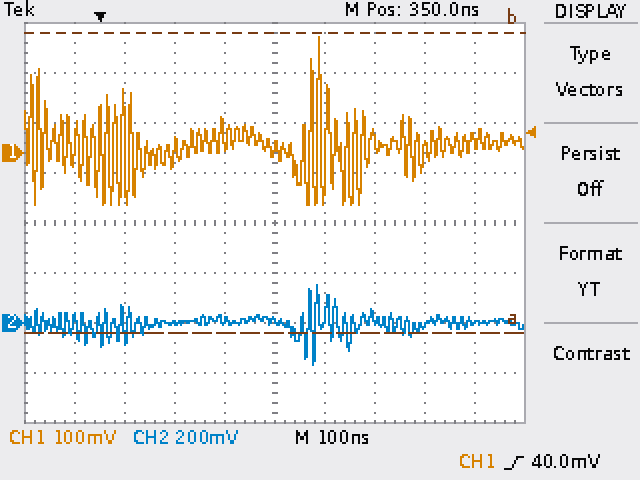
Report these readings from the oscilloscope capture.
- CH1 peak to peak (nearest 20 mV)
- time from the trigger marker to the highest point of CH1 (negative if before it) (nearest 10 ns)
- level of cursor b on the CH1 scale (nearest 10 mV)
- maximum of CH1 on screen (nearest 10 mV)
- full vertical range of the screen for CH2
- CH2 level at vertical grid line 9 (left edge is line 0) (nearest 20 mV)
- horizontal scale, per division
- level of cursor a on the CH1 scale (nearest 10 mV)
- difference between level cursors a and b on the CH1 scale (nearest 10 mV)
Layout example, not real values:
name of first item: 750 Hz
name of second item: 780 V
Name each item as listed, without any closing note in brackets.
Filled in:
CH1 peak to peak: 340 mV
time from the trigger marker to the highest point of CH1 (negative if before it): +440 ns
level of cursor b on the CH1 scale: 240 mV
maximum of CH1 on screen: 230 mV
full vertical range of the screen for CH2: 1.6 V
CH2 level at vertical grid line 9 (left edge is line 0): 0 mV
horizontal scale, per division: 100 ns
level of cursor a on the CH1 scale: -360 mV
difference between level cursors a and b on the CH1 scale: 600 mV
